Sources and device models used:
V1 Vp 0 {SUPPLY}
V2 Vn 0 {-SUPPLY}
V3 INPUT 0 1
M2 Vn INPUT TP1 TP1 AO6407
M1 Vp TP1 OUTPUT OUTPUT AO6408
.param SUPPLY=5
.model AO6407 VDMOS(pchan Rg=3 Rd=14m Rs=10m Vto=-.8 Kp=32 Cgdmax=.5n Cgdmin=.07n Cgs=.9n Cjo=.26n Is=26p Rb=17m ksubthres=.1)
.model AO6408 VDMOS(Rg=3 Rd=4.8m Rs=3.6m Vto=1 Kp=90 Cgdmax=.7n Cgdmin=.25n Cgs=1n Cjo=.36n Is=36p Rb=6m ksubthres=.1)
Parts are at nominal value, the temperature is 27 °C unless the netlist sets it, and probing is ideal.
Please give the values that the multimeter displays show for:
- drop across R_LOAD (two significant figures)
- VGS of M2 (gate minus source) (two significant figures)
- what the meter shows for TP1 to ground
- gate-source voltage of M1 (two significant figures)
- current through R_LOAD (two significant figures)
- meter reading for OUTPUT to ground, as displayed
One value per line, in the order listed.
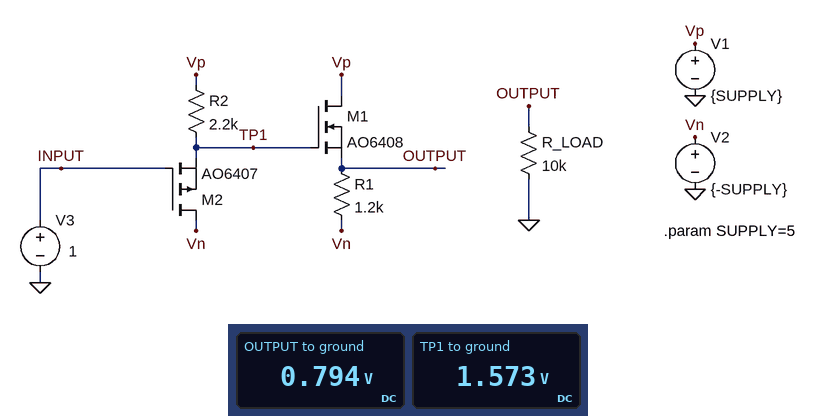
790 mV
-570 mV
1.573 V
780 mV
79 µA
0.794 V
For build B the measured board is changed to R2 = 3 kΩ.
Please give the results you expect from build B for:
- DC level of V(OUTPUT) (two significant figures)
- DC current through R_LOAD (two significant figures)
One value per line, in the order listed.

780 mV
78 µA
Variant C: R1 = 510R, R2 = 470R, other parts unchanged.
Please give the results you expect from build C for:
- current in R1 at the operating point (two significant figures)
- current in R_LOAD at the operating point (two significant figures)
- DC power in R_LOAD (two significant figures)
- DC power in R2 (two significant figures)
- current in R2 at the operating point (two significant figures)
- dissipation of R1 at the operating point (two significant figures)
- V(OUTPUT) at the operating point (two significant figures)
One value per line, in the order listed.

11 mA
83 µA
69 µW
24 mW
7.1 mA
67 mW
830 mV
